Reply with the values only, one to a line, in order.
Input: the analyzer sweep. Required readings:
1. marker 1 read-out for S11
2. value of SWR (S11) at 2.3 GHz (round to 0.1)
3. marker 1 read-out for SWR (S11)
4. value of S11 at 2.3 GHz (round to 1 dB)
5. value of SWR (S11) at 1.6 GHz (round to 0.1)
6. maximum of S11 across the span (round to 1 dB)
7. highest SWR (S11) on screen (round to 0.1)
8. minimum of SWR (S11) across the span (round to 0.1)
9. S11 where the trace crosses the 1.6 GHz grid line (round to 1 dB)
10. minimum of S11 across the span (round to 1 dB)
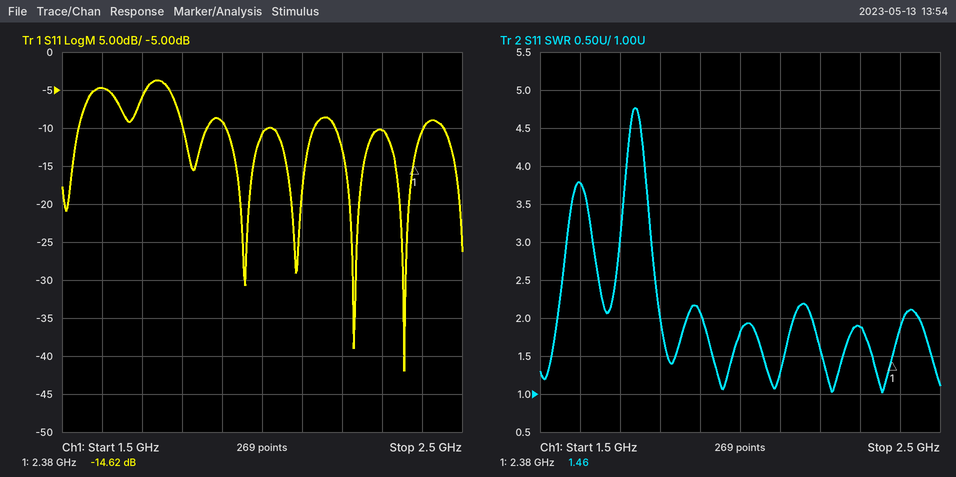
-14.62 dB
1.9
1.46
-10 dB
3.8
-4 dB
4.8
1.0
-5 dB
-42 dB
